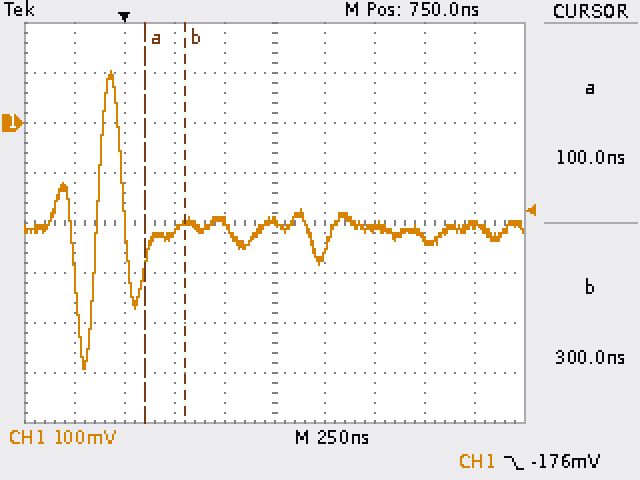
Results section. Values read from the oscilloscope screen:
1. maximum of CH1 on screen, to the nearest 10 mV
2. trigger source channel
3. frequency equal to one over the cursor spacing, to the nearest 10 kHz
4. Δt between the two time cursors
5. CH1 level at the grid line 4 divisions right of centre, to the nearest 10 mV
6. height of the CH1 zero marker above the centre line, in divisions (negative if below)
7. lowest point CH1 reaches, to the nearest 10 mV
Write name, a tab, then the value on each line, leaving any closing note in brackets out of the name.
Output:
maximum of CH1 on screen, to the nearest 10 mV	100 mV
trigger source channel	CH1
frequency equal to one over the cursor spacing, to the nearest 10 kHz	5.00 MHz
Δt between the two time cursors	200 ns
CH1 level at the grid line 4 divisions right of centre, to the nearest 10 mV	-200 mV
height of the CH1 zero marker above the centre line, in divisions	+2.0 div
lowest point CH1 reaches, to the nearest 10 mV	-490 mV
